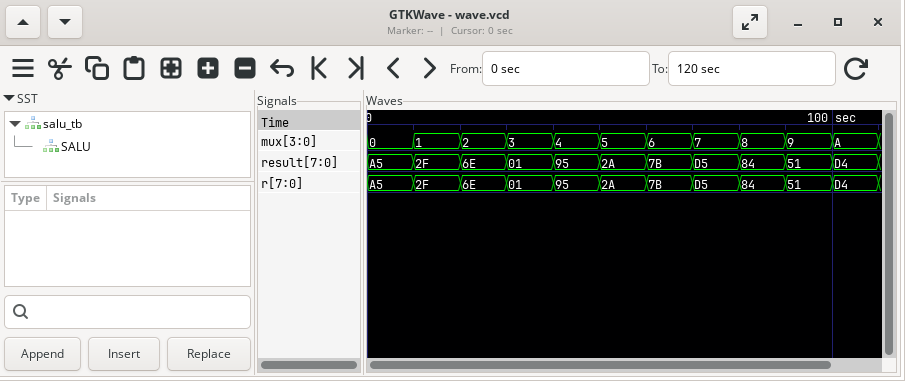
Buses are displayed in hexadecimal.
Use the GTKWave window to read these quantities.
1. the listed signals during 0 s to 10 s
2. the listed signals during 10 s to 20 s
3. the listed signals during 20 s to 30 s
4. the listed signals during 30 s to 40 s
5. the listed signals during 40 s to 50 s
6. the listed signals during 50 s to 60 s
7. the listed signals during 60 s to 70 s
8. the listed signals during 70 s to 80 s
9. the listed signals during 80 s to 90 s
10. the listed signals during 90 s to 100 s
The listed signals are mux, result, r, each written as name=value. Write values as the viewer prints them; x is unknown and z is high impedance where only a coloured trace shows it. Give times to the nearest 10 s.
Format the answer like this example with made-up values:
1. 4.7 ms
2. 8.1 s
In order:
1. mux=0, result=A5, r=A5
2. mux=1, result=2F, r=2F
3. mux=2, result=6E, r=6E
4. mux=3, result=01, r=01
5. mux=4, result=95, r=95
6. mux=5, result=2A, r=2A
7. mux=6, result=7B, r=7B
8. mux=7, result=D5, r=D5
9. mux=8, result=84, r=84
10. mux=9, result=51, r=51
